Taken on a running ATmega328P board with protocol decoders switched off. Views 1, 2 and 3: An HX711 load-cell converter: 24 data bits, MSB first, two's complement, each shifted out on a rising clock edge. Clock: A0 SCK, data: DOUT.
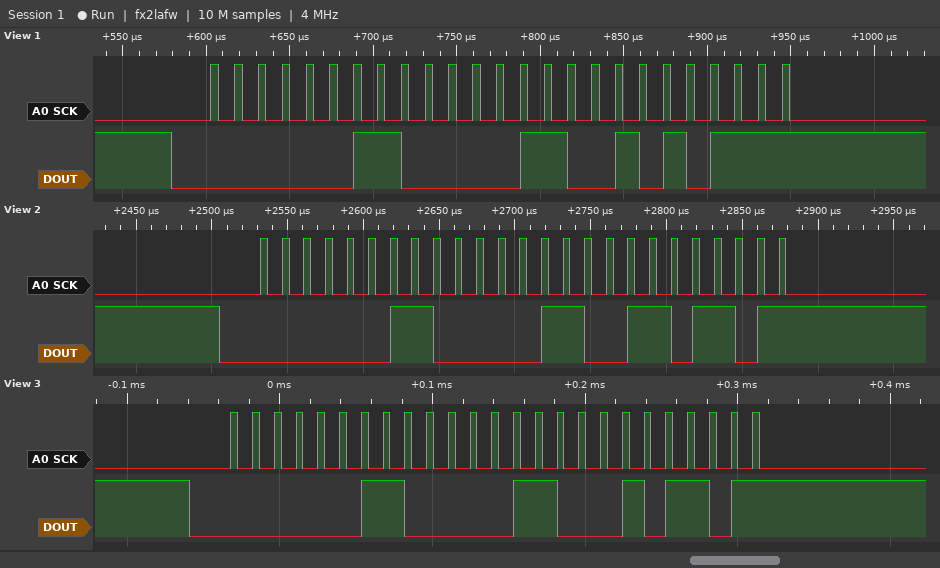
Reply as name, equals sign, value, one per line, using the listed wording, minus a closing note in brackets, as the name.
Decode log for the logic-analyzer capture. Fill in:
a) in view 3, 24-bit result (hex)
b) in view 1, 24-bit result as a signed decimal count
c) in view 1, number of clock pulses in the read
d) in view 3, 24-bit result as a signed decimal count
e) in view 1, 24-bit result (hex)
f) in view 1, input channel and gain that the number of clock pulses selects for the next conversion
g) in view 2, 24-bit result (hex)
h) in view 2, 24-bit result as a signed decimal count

in view 3, 24-bit result = 0x03062D
in view 1, 24-bit result as a signed decimal count = 198231
in view 1, number of clock pulses in the read = 25
in view 3, 24-bit result as a signed decimal count = 198189
in view 1, 24-bit result = 0x030657
in view 1, input channel and gain that the number of clock pulses selects for the next conversion = channel A, gain 128
in view 2, 24-bit result = 0x03066D
in view 2, 24-bit result as a signed decimal count = 198253
